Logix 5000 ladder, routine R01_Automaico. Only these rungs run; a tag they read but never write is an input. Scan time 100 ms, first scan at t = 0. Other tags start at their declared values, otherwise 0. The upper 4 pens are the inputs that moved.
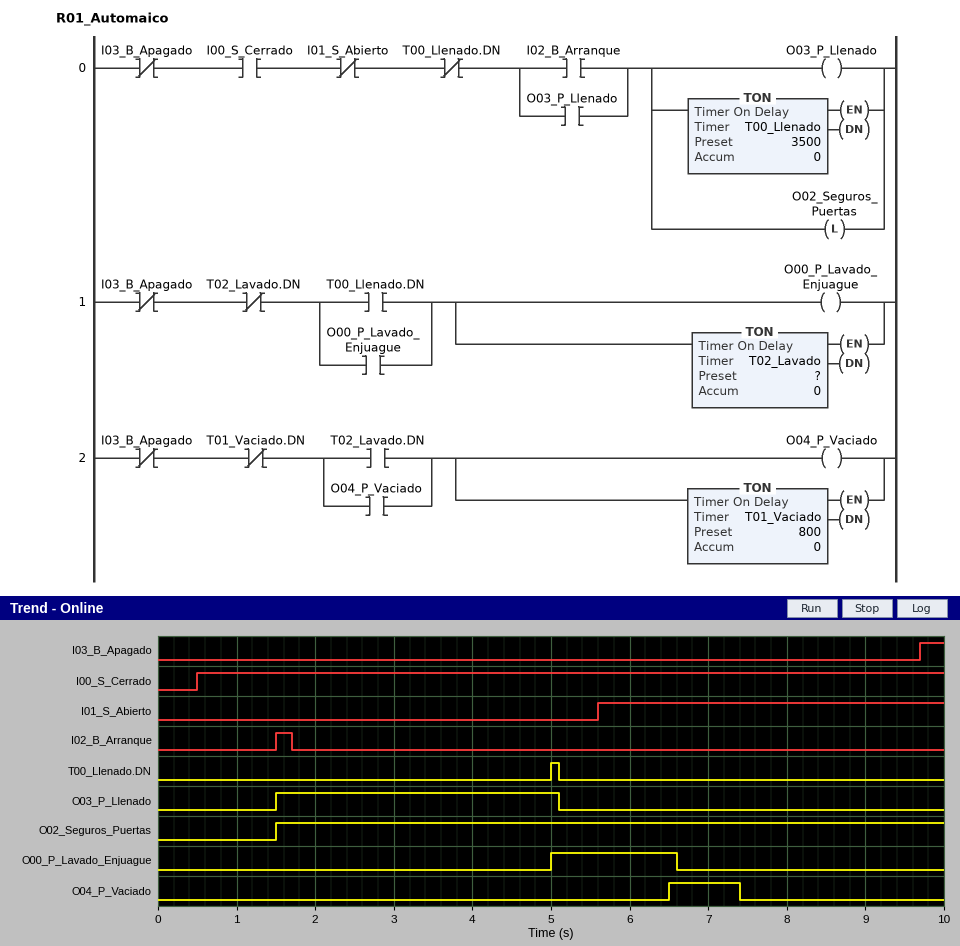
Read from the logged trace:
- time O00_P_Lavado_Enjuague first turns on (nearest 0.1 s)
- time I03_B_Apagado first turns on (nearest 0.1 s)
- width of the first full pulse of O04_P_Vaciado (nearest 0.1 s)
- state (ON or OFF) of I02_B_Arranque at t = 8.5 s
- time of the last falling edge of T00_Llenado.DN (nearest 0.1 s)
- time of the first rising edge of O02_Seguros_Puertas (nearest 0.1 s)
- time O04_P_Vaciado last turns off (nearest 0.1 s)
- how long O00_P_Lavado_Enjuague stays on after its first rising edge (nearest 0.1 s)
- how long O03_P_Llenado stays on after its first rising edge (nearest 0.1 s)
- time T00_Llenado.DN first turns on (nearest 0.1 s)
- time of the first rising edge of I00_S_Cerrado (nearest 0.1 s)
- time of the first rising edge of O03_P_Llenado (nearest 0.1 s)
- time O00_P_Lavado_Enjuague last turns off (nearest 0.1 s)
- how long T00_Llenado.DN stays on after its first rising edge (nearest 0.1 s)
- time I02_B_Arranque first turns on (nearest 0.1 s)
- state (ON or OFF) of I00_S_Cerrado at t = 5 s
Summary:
5.0 s
9.7 s
0.9 s
OFF
5.1 s
1.5 s
7.4 s
1.6 s
3.6 s
5.0 s
0.5 s
1.5 s
6.6 s
0.1 s
1.5 s
ON
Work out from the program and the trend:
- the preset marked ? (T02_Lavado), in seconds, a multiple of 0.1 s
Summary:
1.5 s
